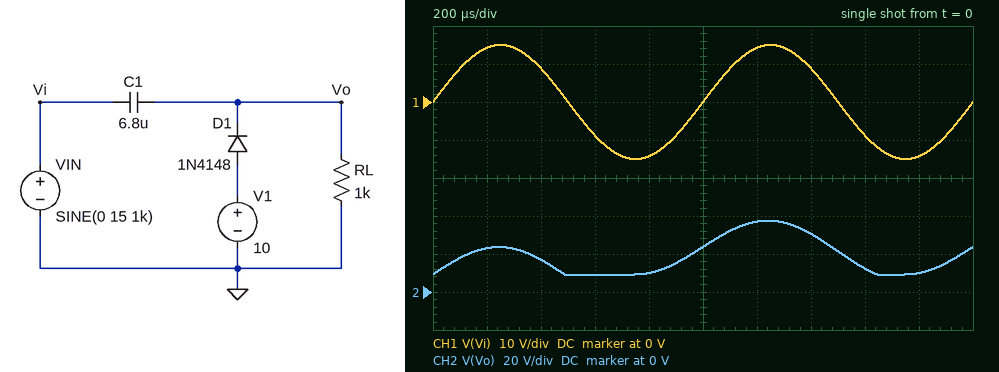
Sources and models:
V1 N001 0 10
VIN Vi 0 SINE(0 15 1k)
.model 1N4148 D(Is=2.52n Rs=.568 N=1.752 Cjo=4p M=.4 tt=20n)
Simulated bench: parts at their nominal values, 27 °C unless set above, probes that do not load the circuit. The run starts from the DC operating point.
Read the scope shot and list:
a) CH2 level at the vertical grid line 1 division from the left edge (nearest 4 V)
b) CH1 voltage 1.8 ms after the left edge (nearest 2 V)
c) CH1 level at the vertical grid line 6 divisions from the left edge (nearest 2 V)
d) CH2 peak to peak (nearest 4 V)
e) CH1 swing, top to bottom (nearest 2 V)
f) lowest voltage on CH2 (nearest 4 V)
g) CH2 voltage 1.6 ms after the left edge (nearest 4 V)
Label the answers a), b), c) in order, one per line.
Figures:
a) 24 V
b) -14 V
c) 14 V
d) 28 V
e) 30 V
f) 8 V
g) 12 V
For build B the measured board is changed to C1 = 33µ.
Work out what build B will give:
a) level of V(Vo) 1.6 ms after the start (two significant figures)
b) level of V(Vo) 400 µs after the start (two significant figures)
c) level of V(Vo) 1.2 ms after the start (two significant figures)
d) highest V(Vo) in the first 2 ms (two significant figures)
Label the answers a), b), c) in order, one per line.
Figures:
a) 15 V
b) 18 V
c) 38 V
d) 39 V
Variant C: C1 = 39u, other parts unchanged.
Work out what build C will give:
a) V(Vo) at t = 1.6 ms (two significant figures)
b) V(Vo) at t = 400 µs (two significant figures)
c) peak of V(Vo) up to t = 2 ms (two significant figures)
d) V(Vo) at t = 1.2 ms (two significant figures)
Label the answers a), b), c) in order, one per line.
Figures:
a) 15 V
b) 18 V
c) 39 V
d) 38 V
